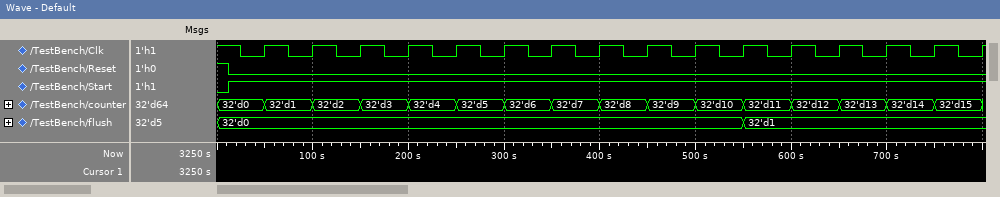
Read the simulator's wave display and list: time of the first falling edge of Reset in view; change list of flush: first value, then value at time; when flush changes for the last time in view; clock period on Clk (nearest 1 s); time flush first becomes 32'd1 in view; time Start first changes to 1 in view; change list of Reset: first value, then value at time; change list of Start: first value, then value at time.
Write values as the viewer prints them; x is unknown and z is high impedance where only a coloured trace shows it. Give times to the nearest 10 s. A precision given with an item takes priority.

10 s
32'd0, 32'd1 at 550 s
550 s
50 s
550 s
10 s
1, 0 at 10 s
0, 1 at 10 s
